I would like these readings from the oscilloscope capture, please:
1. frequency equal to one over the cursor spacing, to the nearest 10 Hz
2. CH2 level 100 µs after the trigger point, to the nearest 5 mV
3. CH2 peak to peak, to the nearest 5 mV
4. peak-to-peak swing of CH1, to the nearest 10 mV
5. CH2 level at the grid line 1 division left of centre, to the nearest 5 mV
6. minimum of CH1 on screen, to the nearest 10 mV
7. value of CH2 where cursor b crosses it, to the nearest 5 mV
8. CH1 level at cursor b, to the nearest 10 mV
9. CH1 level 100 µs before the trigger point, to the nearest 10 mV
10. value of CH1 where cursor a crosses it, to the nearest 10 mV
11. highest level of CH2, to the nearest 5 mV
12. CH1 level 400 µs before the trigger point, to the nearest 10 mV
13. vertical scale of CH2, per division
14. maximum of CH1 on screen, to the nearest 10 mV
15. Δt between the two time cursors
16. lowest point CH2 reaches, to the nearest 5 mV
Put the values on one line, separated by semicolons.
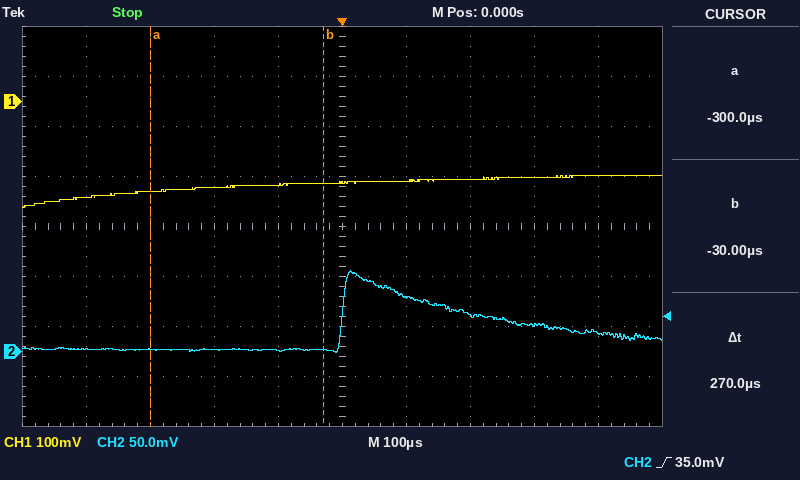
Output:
3.70 kHz; 55 mV; 80 mV; 60 mV; 0 mV; -210 mV; 0 mV; -160 mV; -170 mV; -180 mV; 80 mV; -190 mV; 50 mV; -150 mV; 270 µs; 0 mV
